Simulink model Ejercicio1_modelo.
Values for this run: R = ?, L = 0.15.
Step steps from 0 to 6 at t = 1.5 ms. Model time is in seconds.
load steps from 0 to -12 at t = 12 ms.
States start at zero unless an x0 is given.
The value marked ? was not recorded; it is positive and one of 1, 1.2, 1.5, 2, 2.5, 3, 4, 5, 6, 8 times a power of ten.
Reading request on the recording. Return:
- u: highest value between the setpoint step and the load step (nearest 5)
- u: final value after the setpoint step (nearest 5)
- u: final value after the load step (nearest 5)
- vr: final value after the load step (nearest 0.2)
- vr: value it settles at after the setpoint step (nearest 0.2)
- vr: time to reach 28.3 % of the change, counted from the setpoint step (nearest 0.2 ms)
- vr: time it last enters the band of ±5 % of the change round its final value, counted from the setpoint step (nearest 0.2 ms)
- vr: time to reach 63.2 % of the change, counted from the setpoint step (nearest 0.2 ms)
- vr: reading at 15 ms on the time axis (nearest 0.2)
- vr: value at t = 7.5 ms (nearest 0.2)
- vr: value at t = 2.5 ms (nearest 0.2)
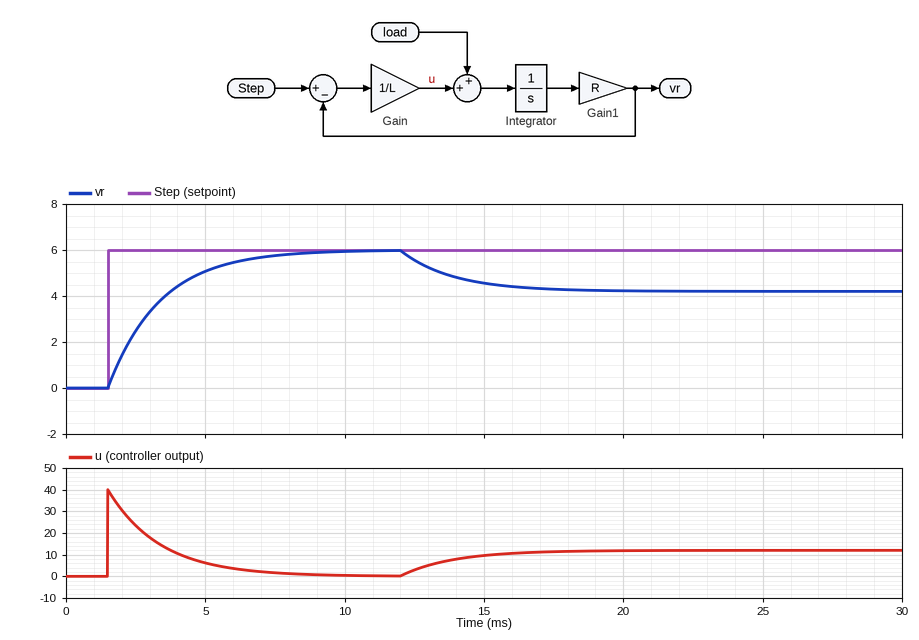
40
0
10
4.2
6.0
0.6 ms
5.6 ms
1.8 ms
4.6
5.8
2.4
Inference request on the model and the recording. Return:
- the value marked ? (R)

80
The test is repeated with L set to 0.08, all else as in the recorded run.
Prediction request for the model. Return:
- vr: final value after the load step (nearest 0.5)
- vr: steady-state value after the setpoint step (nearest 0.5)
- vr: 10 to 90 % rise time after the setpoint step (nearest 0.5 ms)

5.0
6.0
2.0 ms
